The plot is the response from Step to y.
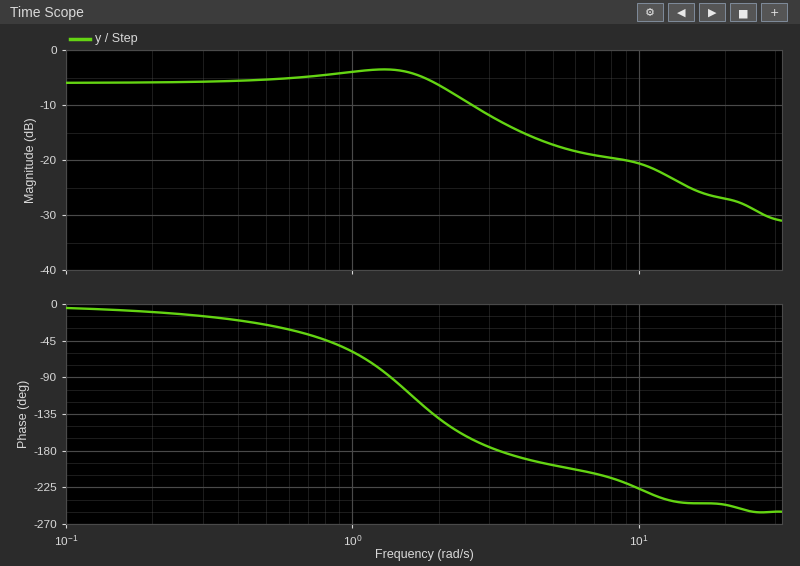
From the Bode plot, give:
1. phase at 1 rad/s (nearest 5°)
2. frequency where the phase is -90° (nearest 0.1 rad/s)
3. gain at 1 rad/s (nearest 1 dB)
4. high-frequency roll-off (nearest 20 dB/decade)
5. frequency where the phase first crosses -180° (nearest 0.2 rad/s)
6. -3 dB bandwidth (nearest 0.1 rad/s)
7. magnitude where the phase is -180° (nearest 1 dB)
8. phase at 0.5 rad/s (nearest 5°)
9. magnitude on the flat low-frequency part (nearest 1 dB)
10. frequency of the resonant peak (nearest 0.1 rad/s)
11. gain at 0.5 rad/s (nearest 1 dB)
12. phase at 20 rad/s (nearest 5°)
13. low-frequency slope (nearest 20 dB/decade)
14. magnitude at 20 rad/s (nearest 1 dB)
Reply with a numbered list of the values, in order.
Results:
1. -60°
2. 1.4 rad/s
3. -4 dB
4. -20 dB/decade
5. 3.2 rad/s
6. 2.4 rad/s
7. -13 dB
8. -25°
9. -6 dB
10. 1.3 rad/s
11. -5 dB
12. -245°
13. 0 dB/decade
14. -27 dB
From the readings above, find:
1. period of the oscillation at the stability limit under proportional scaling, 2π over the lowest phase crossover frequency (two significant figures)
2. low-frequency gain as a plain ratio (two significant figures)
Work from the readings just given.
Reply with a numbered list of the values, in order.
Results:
1. 2.0 s
2. 0.50
